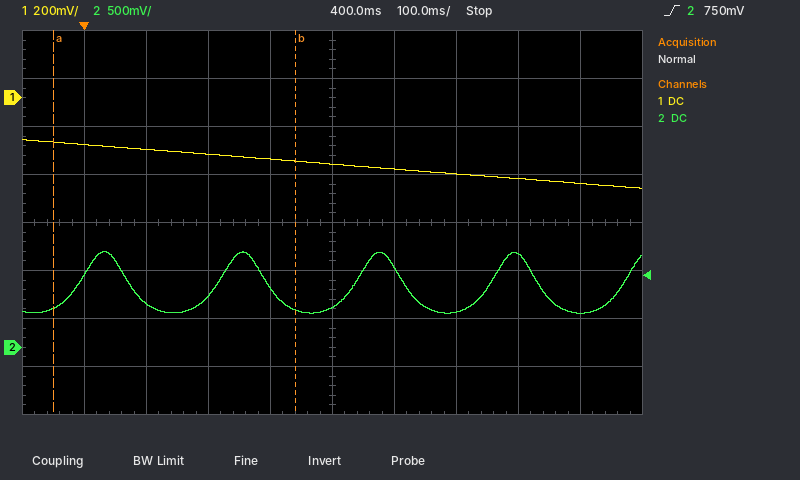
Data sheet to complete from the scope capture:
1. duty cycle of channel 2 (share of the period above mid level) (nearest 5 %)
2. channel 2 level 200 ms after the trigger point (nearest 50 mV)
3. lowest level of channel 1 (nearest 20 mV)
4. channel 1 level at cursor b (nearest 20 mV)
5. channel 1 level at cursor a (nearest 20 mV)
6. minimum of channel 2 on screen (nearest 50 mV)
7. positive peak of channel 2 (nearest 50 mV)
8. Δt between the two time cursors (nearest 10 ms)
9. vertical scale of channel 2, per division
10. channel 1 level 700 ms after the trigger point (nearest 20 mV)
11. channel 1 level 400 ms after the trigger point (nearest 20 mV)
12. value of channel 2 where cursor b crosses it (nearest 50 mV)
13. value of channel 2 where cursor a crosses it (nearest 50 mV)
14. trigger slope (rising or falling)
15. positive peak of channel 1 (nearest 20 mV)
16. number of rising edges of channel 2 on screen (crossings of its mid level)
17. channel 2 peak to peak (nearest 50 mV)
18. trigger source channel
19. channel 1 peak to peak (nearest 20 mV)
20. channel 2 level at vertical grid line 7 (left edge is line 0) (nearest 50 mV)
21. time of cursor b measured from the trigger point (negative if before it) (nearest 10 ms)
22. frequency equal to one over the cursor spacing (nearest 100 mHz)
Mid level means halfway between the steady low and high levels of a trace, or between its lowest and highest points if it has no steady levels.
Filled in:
35 %
550 mV
-380 mV
-260 mV
-180 mV
350 mV
1.00 V
390 ms
500 mV
-340 mV
-280 mV
400 mV
400 mV
rising
-180 mV
5
650 mV
channel 2
200 mV
350 mV
+340 ms
2.6 Hz
